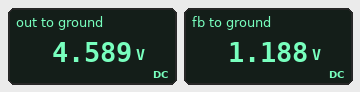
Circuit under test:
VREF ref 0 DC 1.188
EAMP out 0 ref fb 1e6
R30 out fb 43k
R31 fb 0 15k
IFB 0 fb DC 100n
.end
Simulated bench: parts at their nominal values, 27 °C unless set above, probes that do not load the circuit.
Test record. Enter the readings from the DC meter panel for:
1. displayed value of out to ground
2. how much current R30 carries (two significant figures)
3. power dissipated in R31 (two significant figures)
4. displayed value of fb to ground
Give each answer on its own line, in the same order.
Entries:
4.589 V
79 µA
94 µW
1.188 V
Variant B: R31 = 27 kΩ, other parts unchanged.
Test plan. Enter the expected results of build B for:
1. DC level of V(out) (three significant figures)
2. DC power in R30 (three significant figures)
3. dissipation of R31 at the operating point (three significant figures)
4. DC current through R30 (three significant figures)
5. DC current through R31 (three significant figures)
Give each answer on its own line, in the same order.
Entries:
3.08 V
82.9 µW
52.3 µW
43.9 µA
44.0 µA
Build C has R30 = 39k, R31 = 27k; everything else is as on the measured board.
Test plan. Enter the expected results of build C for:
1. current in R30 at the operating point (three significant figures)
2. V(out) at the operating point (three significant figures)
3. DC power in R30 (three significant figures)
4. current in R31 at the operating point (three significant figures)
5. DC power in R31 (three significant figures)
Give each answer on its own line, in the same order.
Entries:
43.9 µA
2.90 V
75.2 µW
44.0 µA
52.3 µW
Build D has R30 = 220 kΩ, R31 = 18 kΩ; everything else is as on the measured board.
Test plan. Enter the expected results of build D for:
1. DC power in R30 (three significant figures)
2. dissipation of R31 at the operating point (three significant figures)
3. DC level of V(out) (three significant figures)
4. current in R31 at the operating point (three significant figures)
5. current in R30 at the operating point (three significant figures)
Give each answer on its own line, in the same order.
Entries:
955 µW
78.4 µW
15.7 V
66.0 µA
65.9 µA
